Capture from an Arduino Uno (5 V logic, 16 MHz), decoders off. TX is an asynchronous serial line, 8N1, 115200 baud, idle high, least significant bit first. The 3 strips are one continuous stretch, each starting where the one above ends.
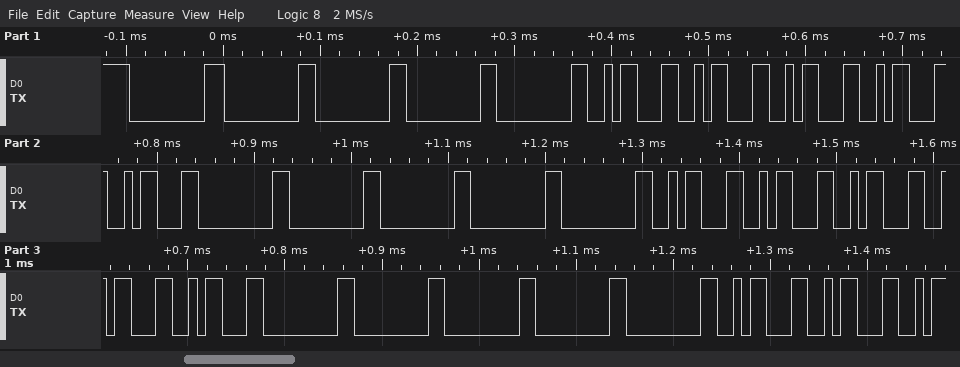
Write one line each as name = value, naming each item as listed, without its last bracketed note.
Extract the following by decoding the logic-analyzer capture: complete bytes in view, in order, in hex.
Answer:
complete bytes in view, in order, in hex = 00 00 00 00 00 1A 1A 1A 1A 1A 00 00 00 00 00 1A 1A 1A 1A 1A 00 00 00 00 00 1A 1A
